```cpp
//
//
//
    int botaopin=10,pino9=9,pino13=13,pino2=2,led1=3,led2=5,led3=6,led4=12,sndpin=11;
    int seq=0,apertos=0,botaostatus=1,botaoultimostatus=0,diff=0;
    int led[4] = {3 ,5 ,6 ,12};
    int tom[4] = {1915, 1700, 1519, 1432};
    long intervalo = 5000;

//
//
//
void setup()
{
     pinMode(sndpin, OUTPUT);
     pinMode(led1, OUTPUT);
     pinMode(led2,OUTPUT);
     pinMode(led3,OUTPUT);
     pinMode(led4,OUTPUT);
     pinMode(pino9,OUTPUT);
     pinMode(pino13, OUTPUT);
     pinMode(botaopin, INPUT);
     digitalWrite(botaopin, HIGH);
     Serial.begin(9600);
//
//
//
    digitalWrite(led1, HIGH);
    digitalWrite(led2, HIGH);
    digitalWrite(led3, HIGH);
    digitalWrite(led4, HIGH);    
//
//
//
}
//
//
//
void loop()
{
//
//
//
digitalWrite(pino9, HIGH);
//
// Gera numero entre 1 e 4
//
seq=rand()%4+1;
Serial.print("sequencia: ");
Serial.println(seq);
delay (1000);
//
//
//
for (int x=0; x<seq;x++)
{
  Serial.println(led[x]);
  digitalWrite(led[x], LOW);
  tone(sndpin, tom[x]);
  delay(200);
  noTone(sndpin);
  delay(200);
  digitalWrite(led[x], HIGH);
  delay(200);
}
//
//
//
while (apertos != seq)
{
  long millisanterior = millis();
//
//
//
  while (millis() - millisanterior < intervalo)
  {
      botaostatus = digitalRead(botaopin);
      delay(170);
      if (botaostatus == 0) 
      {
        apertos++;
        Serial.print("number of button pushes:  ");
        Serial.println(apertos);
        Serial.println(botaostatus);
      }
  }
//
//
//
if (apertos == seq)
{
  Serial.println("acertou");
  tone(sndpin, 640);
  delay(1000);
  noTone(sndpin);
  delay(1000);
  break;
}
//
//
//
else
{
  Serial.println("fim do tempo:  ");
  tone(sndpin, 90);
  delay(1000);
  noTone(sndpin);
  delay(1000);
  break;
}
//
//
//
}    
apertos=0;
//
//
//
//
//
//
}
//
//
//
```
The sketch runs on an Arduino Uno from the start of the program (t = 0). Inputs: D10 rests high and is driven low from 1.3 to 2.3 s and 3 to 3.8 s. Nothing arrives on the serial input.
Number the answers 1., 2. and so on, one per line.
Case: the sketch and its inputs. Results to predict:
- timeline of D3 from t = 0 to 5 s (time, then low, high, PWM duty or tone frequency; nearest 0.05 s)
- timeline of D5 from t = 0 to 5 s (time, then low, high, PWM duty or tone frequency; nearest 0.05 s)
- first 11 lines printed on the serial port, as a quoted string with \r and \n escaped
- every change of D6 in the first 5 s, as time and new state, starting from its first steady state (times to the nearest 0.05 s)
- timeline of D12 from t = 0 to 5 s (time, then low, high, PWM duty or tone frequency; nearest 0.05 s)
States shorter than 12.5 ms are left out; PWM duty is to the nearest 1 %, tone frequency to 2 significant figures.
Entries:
1. 0 s high; 1 s low; 1.4 s high
2. 0 s high; 1.6 s low; 2 s high
3. "sequencia: 4\r\n3\r\n5\r\n6\r\n12\r\nnumber of button pushes:  1\r\n0\r\nnumber of button pushes:  2\r\n0\r\nnumber of button pushes:  3\r\n0\r\n"
4. 0 s high; 2.2 s low; 2.6 s high
5. 0 s high; 2.8 s low; 3.2 s high
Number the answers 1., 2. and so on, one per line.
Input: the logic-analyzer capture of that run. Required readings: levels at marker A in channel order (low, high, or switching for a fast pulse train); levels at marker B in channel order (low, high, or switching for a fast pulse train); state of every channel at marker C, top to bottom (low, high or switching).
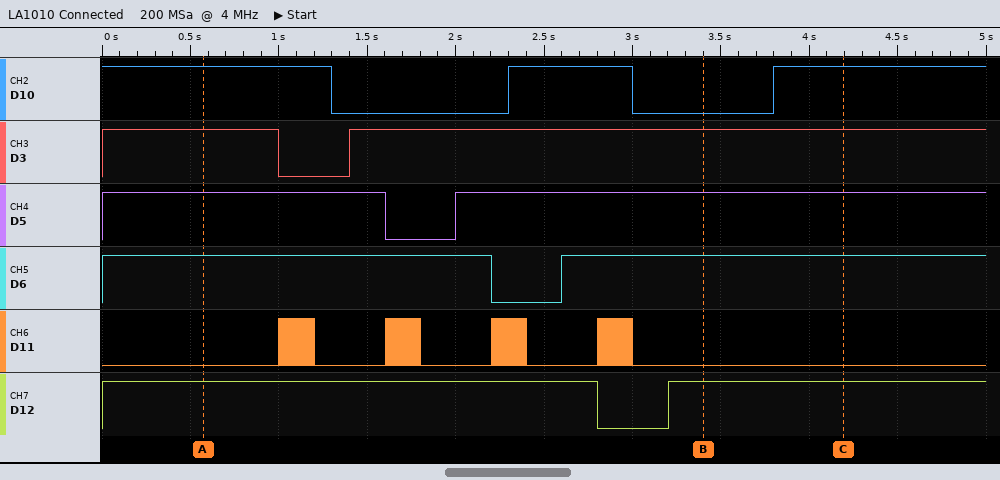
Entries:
1. D10 high, D3 high, D5 high, D6 high, D11 low, D12 high
2. D10 low, D3 high, D5 high, D6 high, D11 low, D12 high
3. D10 high, D3 high, D5 high, D6 high, D11 low, D12 high
